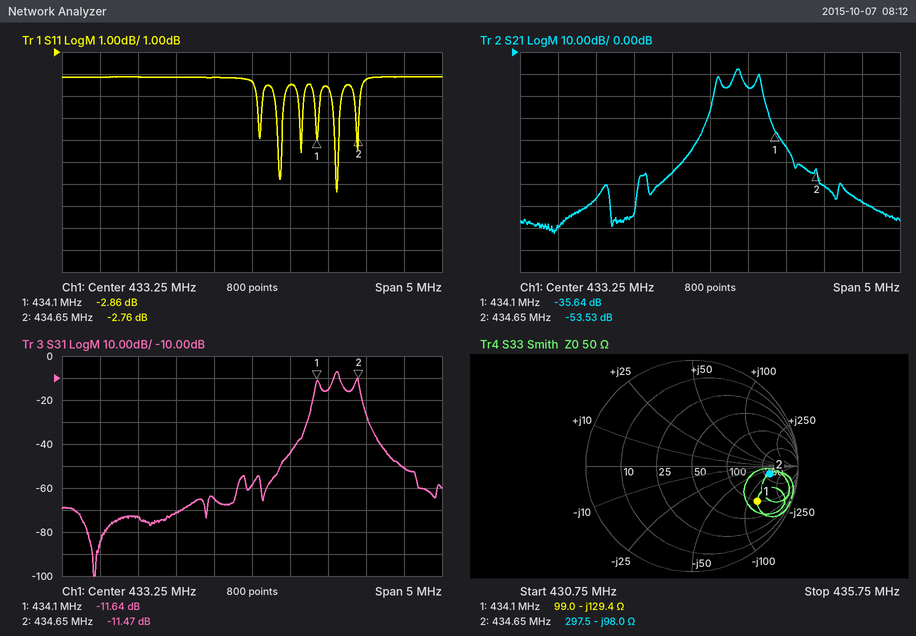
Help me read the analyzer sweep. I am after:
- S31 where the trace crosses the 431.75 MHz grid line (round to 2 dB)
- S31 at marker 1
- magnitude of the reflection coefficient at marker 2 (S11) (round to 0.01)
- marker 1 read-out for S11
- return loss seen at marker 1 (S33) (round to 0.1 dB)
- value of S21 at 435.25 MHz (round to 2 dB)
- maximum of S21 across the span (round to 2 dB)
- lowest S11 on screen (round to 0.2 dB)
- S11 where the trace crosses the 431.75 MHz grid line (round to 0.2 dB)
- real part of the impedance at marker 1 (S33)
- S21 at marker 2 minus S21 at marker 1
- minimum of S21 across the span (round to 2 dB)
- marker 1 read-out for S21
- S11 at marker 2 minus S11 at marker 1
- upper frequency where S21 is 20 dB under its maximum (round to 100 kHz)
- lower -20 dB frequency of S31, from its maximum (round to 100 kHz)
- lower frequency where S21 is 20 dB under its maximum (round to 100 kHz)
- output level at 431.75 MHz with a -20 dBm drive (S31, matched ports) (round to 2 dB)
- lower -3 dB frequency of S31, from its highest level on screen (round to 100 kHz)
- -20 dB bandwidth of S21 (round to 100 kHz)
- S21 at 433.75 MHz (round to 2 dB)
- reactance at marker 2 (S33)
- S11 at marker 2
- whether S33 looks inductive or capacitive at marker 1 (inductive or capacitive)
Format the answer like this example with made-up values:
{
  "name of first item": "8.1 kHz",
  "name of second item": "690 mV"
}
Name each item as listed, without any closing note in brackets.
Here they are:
{
  "S31 where the trace crosses the 431.75 MHz grid line": "-74 dB",
  "S31 at marker 1": "-11.64 dB",
  "magnitude of the reflection coefficient at marker 2 (S11)": "0.73",
  "marker 1 read-out for S11": "-2.86 dB",
  "return loss seen at marker 1 (S33)": "3.1 dB",
  "value of S21 at 435.25 MHz": "-68 dB",
  "maximum of S21 across the span": "-8 dB",
  "lowest S11 on screen": "-5.4 dB",
  "S11 where the trace crosses the 431.75 MHz grid line": "-0.2 dB",
  "real part of the impedance at marker 1": "99.0 Ω",
  "S21 at marker 2 minus S21 at marker 1": "-17.89 dB",
  "minimum of S21 across the span": "-82 dB",
  "marker 1 read-out for S21": "-35.64 dB",
  "S11 at marker 2 minus S11 at marker 1": "0.10 dB",
  "upper frequency where S21 is 20 dB under its maximum": "434.0 MHz",
  "lower -20 dB frequency of S31, from its maximum": "434.0 MHz",
  "lower frequency where S21 is 20 dB under its maximum": "433.2 MHz",
  "output level at 431.75 MHz with a -20 dBm drive (S31, matched ports)": "-94 dBm",
  "lower -3 dB frequency of S31, from its highest level on screen": "434.3 MHz",
  "-20 dB bandwidth of S21": "800 kHz",
  "S21 at 433.75 MHz": "-16 dB",
  "reactance at marker 2": "-98.0 Ω",
  "S11 at marker 2": "-2.76 dB",
  "whether S33 looks inductive or capacitive at marker 1": "capacitive"
}
